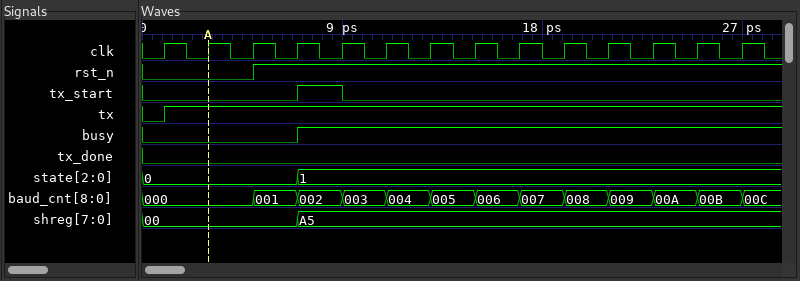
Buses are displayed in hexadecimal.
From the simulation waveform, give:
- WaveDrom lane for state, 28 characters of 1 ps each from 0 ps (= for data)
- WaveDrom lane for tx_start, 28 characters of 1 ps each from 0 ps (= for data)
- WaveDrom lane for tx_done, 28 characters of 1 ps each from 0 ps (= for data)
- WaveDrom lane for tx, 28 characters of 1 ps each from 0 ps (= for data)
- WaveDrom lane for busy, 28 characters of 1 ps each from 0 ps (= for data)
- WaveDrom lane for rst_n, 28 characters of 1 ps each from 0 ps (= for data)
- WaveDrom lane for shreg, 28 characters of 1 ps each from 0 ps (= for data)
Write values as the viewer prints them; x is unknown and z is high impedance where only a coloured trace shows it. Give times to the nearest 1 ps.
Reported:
{name: 'state', wave: '=......=....................', data: '0 1'}
{name: 'tx_start', wave: '0......1.0..................'}
{name: 'tx_done', wave: '0...........................'}
{name: 'tx', wave: '01..........................'}
{name: 'busy', wave: '0......1....................'}
{name: 'rst_n', wave: '0....1......................'}
{name: 'shreg', wave: '=......=....................', data: '00 A5'}
